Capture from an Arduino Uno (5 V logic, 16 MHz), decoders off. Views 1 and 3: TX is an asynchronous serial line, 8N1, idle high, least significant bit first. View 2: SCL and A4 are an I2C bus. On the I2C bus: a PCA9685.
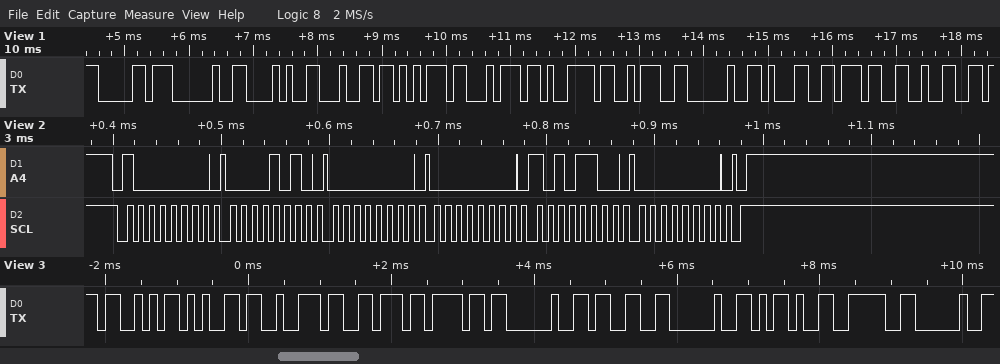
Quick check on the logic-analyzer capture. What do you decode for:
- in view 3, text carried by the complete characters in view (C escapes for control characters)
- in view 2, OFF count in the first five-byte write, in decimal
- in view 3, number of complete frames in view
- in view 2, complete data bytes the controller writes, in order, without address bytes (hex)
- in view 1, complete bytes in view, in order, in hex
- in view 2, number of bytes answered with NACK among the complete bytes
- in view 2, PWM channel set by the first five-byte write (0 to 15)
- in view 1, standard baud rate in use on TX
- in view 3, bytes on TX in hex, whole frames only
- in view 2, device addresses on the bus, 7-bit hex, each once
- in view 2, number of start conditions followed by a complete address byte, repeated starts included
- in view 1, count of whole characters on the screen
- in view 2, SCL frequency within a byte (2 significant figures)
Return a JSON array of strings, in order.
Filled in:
["\"Servo 3 -> \"", "172", "11", "0A 00 00 AC 00", "B0 20 28 64 75 74 79 3A 20 31 37 32", "0", "1", "9600 baud", "53 65 72 76 6F 20 33 20 2D 3E 20", "0x40", "1", "12", "100 kHz"]
